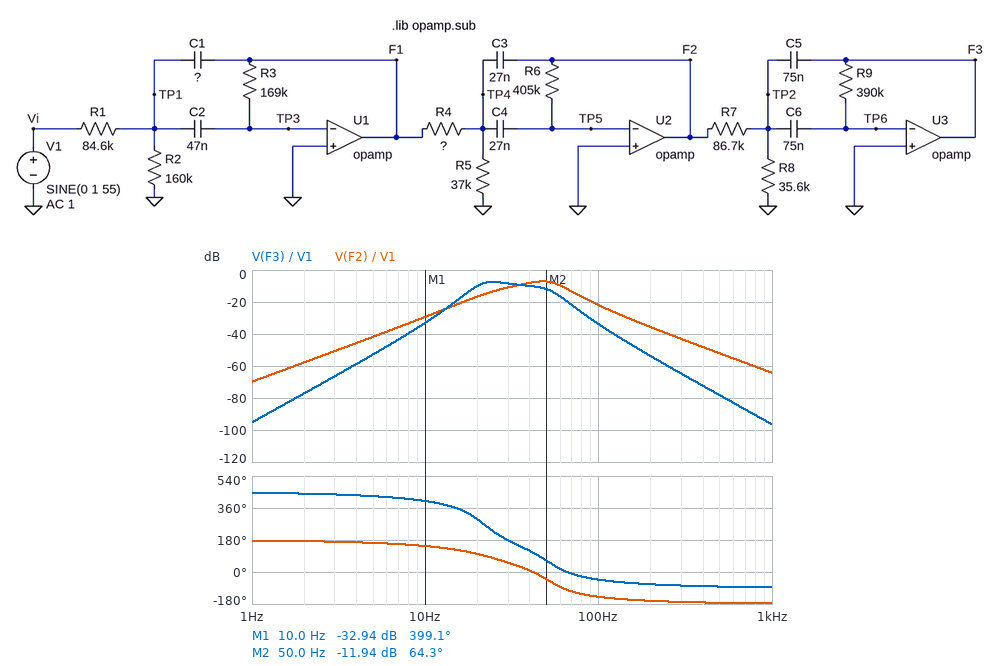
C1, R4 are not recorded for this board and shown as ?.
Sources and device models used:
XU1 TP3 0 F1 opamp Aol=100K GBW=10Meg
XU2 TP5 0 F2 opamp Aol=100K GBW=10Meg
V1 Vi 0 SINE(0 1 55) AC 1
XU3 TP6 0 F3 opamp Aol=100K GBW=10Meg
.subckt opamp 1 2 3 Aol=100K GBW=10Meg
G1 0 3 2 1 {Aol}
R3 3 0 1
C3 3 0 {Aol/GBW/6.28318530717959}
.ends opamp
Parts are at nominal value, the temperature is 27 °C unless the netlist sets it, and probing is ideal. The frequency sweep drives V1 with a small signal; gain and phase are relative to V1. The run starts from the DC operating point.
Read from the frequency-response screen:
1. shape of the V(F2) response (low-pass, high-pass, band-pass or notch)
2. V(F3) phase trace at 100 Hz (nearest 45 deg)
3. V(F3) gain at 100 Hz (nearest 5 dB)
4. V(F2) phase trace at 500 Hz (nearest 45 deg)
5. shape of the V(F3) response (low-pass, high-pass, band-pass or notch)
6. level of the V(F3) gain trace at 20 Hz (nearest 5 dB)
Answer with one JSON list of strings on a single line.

["band-pass", "-45 deg", "-35 dB", "-180 deg", "band-pass", "-10 dB"]
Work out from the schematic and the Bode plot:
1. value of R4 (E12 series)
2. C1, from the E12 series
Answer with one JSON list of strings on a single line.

["220 kΩ", "82 nF"]
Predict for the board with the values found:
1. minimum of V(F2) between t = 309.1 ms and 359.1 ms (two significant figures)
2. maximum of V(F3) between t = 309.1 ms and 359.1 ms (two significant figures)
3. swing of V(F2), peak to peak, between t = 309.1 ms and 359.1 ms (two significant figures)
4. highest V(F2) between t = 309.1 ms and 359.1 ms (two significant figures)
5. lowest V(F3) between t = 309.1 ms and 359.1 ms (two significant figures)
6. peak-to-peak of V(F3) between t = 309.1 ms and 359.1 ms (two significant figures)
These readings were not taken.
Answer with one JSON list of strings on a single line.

["-390 mV", "200 mV", "790 mV", "390 mV", "-200 mV", "400 mV"]
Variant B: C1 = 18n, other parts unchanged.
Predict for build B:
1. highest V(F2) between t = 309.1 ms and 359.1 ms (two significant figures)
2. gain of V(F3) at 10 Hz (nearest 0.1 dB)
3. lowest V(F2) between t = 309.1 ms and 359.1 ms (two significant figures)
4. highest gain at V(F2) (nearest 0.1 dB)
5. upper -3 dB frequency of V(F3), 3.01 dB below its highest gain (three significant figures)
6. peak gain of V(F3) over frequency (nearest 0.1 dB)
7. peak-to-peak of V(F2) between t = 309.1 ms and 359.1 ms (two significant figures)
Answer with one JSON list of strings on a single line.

["1.3 V", "-33.2 dB", "-1.3 V", "2.4 dB", "60.2 Hz", "-2.4 dB", "2.6 V"]
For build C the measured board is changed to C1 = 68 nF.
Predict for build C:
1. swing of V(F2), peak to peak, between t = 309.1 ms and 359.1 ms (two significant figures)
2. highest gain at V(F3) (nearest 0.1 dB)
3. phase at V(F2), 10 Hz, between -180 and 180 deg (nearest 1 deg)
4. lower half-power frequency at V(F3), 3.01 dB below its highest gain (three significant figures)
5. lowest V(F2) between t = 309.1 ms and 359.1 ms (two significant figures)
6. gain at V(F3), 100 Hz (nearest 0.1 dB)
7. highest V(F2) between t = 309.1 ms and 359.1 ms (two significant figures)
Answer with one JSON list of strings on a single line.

["960 mV", "-6.8 dB", "149 deg", "19.8 Hz", "-480 mV", "-32.2 dB", "480 mV"]
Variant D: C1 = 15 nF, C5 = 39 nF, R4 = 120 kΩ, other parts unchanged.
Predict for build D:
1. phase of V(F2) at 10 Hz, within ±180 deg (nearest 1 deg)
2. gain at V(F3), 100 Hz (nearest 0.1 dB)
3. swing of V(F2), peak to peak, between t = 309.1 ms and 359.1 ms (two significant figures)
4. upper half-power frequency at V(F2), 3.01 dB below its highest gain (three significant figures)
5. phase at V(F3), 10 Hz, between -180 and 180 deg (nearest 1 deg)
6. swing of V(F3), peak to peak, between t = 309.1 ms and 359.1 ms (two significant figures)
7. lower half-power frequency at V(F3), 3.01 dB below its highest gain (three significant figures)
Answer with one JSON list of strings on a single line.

["162 deg", "-7.9 dB", "5.0 V", "71.2 Hz", "60 deg", "5.6 V", "32.1 Hz"]
